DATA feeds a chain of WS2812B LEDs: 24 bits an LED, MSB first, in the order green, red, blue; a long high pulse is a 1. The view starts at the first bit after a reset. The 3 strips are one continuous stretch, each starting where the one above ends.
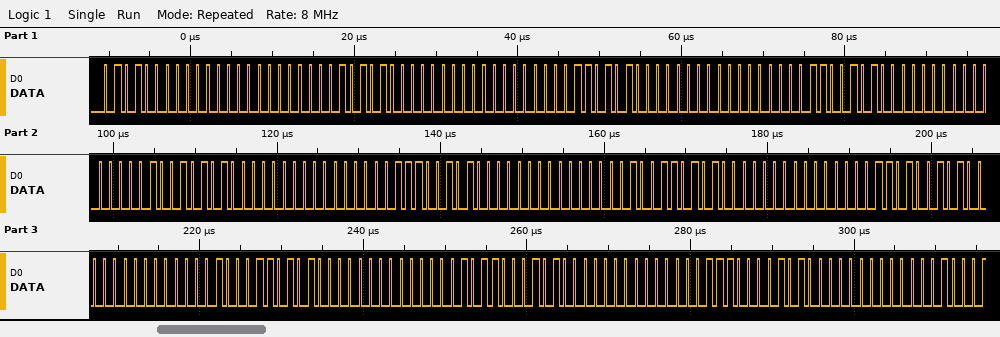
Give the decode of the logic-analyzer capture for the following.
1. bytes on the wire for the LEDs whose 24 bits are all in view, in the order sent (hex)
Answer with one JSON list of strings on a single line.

["50 00 01 50 00 03 50 00 06 50 00 09 50 00 0E 50 00 13 50 00 1A 50 00 23 50 00 2C 50 00 38"]
